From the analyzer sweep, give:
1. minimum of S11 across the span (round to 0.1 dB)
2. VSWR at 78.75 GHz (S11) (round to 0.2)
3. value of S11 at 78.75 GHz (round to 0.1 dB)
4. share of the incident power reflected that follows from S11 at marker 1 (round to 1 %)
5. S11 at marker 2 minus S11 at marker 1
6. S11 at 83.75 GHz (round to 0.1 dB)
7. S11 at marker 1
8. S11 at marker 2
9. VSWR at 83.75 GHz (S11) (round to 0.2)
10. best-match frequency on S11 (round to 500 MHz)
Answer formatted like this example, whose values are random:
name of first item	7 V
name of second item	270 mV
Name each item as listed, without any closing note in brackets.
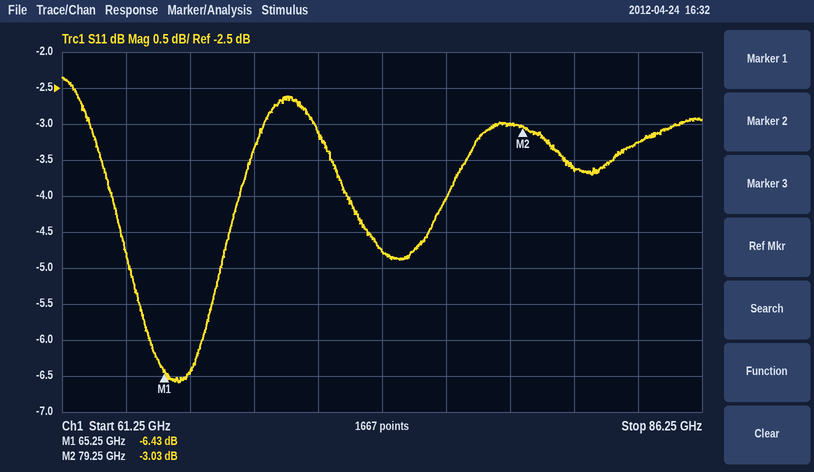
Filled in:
minimum of S11 across the span	-6.6 dB
VSWR at 78.75 GHz (S11)	5.8
value of S11 at 78.75 GHz	-3.0 dB
share of the incident power reflected that follows from S11 at marker 1	23 %
S11 at marker 2 minus S11 at marker 1	3.40 dB
S11 at 83.75 GHz	-3.3 dB
S11 at marker 1	-6.43 dB
S11 at marker 2	-3.03 dB
VSWR at 83.75 GHz (S11)	5.4
best-match frequency on S11	66.0 GHz
